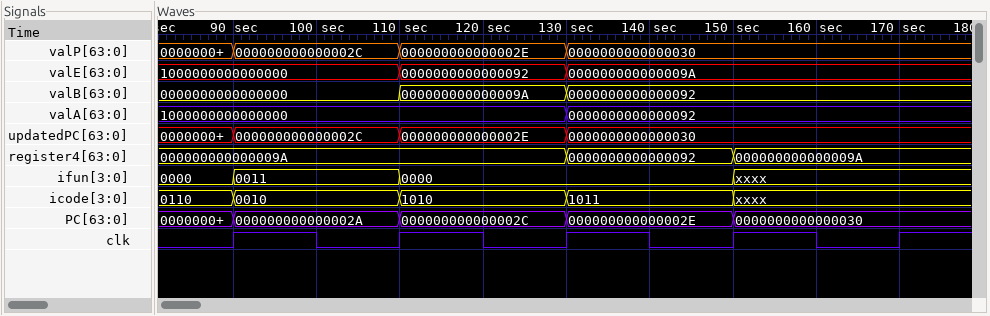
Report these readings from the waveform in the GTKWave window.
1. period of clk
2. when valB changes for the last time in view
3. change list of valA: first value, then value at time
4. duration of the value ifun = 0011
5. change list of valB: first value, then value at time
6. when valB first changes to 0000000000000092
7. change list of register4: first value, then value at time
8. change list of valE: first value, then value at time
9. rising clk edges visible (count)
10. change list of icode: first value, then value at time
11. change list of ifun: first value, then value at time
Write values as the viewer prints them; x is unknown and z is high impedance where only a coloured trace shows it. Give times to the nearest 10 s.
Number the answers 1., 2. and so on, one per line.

1. 20 s
2. 130 s
3. 1000000000000000, 0000000000000092 at 130 s
4. 20 s
5. 0000000000000000, 000000000000009A at 110 s, 0000000000000092 at 130 s
6. 130 s
7. 000000000000009A, 0000000000000092 at 130 s, 000000000000009A at 150 s
8. 1000000000000000, 0000000000000092 at 110 s, 000000000000009A at 130 s
9. 5
10. 0110, 0010 at 90 s, 1010 at 110 s, 1011 at 130 s, xxxx at 150 s
11. 0000, 0011 at 90 s, 0000 at 110 s, xxxx at 150 s
